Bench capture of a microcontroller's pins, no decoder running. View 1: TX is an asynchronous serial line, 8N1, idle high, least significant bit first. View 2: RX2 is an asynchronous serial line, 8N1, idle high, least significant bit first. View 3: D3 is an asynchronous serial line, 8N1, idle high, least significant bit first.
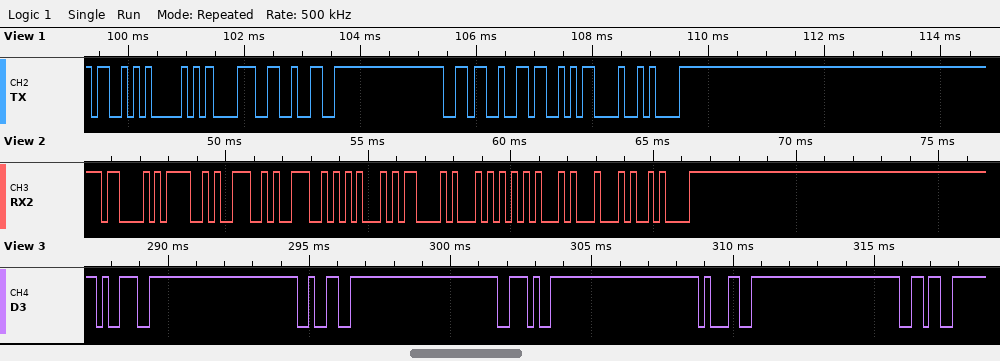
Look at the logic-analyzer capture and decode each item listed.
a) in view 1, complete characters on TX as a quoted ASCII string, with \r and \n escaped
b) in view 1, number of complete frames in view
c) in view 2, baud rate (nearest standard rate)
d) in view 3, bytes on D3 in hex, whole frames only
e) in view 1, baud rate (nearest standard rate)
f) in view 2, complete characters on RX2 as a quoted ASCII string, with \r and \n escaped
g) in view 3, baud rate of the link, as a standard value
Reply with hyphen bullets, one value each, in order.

- "SP8266\r\n"
- 8
- 4800 baud
- 0x39 0x32 0x2E 0x31 0x36
- 9600 baud
- "CONNECTED\n"
- 4800 baud
